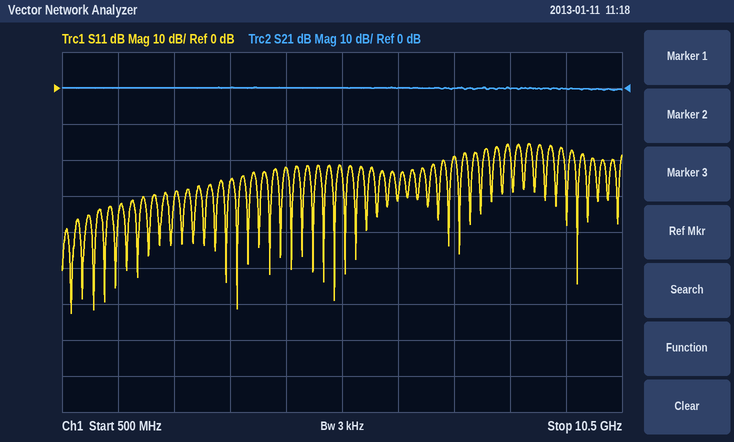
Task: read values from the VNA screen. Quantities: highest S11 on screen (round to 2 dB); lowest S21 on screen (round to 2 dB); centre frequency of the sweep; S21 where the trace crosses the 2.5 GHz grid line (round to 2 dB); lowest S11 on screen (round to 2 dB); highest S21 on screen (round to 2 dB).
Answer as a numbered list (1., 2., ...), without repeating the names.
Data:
1. -16 dB
2. 0 dB
3. 5.5 GHz
4. 0 dB
5. -62 dB
6. 0 dB
